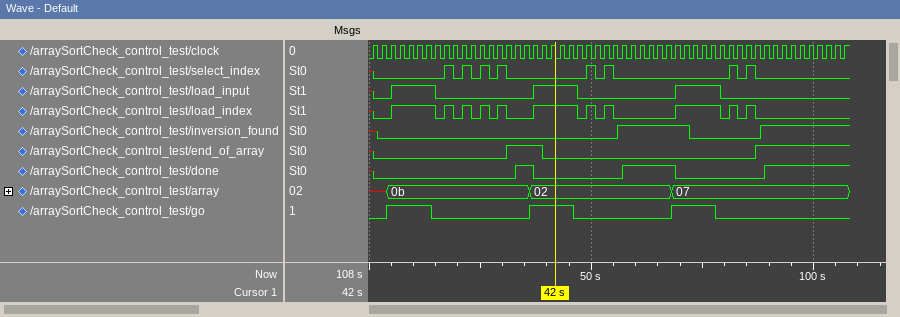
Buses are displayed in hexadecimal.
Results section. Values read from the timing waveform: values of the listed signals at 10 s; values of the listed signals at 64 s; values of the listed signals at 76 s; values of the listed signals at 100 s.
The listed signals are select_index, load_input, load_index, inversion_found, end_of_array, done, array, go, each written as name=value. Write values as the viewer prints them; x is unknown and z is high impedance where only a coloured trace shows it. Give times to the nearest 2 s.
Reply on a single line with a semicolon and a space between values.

select_index=0, load_input=1, load_index=1, inversion_found=0, end_of_array=0, done=0, array=0b, go=1; select_index=0, load_input=0, load_index=0, inversion_found=1, end_of_array=0, done=1, array=02, go=0; select_index=0, load_input=1, load_index=1, inversion_found=0, end_of_array=0, done=0, array=07, go=1; select_index=0, load_input=0, load_index=0, inversion_found=1, end_of_array=1, done=1, array=07, go=0
